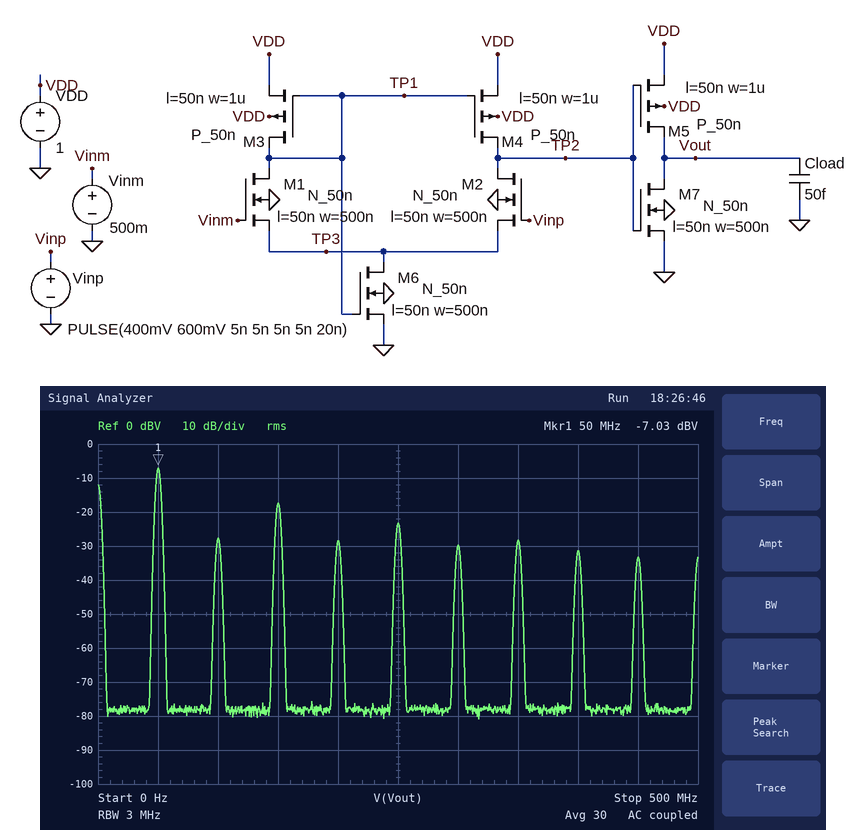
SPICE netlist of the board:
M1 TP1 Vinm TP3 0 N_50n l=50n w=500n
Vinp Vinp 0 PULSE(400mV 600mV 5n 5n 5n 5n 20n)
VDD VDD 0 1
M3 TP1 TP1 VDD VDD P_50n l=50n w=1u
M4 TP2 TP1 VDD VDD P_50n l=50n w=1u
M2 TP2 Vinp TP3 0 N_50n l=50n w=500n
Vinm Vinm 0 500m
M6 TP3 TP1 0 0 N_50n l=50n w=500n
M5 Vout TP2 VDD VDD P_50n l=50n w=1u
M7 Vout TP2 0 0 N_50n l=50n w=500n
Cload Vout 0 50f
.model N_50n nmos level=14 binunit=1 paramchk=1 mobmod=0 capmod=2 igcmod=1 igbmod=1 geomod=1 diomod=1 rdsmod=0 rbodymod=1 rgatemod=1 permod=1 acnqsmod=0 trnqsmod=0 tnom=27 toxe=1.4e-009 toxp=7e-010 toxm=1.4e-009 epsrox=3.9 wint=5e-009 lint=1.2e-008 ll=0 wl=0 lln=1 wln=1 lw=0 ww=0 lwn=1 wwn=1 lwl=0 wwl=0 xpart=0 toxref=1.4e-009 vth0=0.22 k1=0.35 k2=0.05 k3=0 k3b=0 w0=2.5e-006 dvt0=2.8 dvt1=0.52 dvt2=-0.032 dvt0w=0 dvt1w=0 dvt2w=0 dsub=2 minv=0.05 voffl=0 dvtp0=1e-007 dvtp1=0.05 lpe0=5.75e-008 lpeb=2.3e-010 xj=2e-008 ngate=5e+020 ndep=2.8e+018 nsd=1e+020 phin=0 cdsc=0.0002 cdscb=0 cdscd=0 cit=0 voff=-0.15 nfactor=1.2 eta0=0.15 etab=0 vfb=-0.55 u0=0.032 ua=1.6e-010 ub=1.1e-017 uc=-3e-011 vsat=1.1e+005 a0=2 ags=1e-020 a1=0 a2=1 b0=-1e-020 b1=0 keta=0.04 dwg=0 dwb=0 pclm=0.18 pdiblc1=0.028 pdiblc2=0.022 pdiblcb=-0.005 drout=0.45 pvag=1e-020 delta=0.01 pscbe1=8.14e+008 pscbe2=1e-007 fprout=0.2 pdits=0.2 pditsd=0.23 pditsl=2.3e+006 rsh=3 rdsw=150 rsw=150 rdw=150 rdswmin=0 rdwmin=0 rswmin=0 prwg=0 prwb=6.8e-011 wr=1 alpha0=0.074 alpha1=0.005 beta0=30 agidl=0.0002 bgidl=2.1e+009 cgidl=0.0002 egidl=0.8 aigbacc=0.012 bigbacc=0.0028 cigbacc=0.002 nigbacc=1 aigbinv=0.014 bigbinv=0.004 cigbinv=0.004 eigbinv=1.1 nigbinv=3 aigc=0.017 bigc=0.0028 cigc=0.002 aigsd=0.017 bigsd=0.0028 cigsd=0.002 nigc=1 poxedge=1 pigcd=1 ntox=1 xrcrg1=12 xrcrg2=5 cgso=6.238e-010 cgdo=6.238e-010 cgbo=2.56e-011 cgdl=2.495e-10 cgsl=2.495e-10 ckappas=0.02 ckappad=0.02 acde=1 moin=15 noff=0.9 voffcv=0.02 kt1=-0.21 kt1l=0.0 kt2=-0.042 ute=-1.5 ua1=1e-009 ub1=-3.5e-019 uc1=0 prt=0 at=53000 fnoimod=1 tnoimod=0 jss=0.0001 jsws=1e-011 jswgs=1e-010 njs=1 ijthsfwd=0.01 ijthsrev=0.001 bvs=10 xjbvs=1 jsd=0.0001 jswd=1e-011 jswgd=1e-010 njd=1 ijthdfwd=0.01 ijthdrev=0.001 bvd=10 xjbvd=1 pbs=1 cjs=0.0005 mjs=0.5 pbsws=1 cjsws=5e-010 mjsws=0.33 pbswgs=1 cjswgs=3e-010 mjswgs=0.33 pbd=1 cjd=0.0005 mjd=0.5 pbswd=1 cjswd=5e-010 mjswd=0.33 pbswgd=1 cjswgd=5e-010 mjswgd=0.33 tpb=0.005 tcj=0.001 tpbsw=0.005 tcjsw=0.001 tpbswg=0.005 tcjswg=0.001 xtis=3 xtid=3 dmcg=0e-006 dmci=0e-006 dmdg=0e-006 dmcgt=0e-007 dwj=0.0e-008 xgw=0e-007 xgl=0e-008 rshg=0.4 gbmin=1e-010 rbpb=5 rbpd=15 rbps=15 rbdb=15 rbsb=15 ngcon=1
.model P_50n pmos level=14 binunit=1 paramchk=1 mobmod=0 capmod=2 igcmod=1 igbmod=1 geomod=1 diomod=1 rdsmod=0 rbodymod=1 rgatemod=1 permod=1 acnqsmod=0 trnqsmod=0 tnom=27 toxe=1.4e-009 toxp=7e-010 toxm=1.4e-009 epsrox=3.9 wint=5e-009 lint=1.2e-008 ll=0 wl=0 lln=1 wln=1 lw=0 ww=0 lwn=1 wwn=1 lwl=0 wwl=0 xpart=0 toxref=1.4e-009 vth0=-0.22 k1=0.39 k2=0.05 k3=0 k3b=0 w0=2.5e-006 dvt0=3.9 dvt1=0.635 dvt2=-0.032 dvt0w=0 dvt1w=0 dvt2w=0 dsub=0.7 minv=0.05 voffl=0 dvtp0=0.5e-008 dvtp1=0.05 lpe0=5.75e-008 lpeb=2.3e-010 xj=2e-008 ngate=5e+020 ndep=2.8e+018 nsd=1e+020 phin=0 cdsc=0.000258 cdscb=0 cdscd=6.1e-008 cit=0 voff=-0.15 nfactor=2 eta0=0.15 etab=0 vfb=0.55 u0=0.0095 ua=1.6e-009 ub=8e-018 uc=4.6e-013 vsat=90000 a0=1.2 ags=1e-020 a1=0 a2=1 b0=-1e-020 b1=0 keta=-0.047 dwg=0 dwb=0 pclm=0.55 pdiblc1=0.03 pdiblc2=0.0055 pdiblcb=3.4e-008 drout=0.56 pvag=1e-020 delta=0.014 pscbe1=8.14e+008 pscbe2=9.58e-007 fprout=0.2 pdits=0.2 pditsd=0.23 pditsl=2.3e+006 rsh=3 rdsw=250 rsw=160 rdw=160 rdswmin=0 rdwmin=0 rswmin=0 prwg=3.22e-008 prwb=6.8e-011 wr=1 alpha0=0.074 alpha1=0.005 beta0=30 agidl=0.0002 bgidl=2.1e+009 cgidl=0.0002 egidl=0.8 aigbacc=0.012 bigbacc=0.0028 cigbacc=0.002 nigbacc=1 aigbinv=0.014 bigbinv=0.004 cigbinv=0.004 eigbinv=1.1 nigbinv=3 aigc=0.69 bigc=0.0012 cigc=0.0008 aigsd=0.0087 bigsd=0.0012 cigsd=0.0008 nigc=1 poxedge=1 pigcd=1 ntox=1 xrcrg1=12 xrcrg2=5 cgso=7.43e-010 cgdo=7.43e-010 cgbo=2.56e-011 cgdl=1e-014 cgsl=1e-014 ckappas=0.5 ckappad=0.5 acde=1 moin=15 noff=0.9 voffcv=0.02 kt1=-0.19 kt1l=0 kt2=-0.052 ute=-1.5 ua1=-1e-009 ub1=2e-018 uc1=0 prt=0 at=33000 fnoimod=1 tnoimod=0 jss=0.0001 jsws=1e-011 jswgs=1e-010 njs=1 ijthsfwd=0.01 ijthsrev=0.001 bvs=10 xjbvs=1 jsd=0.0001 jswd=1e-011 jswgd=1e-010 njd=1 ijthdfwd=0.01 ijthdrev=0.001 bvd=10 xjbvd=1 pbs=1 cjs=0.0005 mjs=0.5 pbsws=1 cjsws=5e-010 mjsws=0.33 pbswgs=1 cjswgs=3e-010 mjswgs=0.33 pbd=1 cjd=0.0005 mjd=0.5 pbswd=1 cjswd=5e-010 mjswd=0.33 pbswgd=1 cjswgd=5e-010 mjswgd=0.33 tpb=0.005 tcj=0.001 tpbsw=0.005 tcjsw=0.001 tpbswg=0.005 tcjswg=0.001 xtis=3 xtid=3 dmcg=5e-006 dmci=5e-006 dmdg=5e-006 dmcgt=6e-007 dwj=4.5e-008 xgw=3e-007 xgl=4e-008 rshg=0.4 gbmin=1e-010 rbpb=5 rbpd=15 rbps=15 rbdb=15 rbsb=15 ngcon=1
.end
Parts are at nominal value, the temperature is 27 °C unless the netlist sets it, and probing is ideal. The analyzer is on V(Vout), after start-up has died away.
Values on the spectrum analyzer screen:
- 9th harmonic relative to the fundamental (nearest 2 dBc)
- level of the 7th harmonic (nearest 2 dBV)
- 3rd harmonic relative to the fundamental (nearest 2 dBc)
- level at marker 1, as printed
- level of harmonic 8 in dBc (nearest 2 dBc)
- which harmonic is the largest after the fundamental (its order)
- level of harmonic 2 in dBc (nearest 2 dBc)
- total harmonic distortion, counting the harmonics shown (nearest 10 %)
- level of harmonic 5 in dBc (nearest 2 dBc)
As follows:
-26 dBc
-28 dBV
-10 dBc
-7.03 dBV
-24 dBc
3
-20 dBc
40 %
-16 dBc
